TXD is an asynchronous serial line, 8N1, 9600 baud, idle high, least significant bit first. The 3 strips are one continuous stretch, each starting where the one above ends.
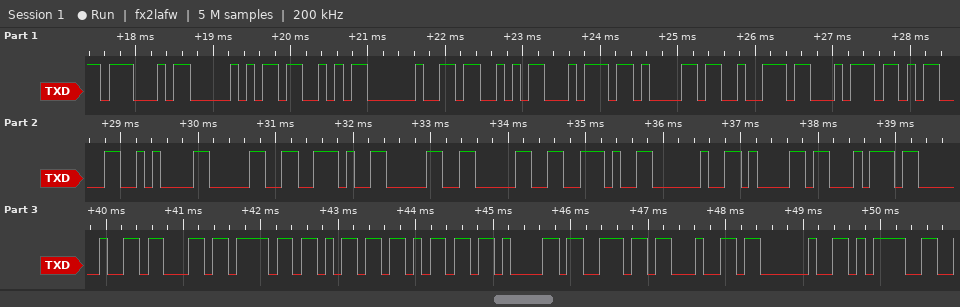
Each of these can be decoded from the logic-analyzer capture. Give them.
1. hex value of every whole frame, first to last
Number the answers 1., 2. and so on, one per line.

1. 0x47 0x50 0x53 0x20 0x53 0x74 0x61 0x72 0x74 0x0D 0x0A 0x30 0x2E 0x30 0x30 0x2E 0x20 0x61 0x74 0x20 0x63 0x6F 0x6D 0x6D 0x61 0x6E 0x64 0x20 0x3D
